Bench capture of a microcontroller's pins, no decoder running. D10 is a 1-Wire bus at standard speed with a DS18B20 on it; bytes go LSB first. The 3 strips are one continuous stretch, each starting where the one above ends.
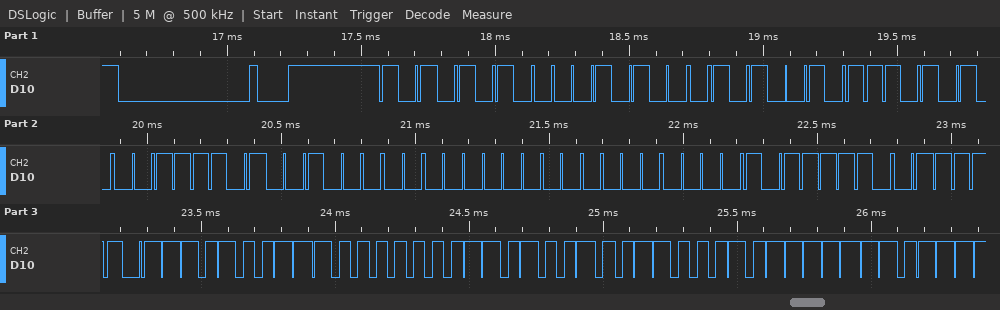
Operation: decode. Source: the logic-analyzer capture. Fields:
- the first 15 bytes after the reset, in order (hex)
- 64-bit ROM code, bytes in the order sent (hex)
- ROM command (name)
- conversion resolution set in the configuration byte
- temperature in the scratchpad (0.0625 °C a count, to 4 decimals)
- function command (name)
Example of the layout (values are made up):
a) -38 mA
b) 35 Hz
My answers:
a) 55 28 4A 57 BC 04 00 00 7D BE CB 01 4B 46 7F
b) 28 4A 57 BC 04 00 00 7D
c) Match ROM
d) 12 bits
e) 28.6875 °C
f) Read Scratchpad
